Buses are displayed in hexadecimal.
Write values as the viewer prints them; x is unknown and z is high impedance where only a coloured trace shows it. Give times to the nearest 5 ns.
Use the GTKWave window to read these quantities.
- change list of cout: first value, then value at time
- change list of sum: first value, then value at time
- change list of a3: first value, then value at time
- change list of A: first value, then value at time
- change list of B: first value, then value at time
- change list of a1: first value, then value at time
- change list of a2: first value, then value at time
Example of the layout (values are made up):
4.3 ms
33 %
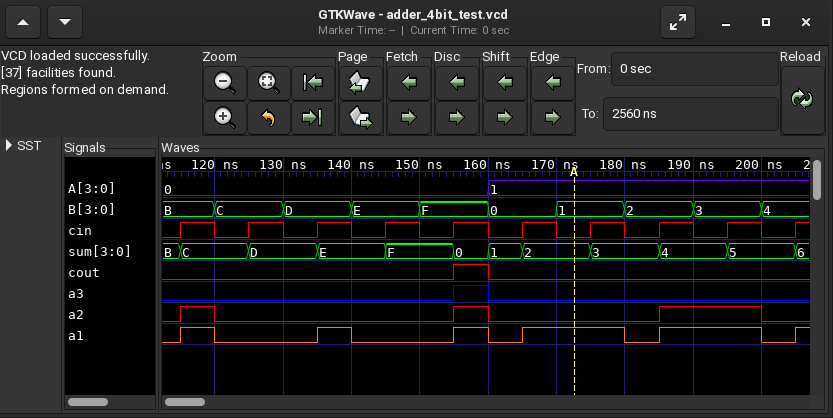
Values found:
0, 1 at 155 ns, 0 at 160 ns
B, C at 115 ns, D at 125 ns, E at 135 ns, F at 145 ns, 0 at 155 ns, 1 at 160 ns, 2 at 165 ns, 3 at 175 ns, 4 at 185 ns, 5 at 195 ns, 6 at 205 ns
0, 1 at 155 ns, 0 at 160 ns
0, 1 at 160 ns
B, C at 120 ns, D at 130 ns, E at 140 ns, F at 150 ns, 0 at 160 ns, 1 at 170 ns, 2 at 180 ns, 3 at 190 ns, 4 at 200 ns
0, 1 at 115 ns, 0 at 120 ns, 1 at 135 ns, 0 at 140 ns, 1 at 155 ns, 0 at 160 ns, 1 at 165 ns, 0 at 180 ns, 1 at 185 ns, 0 at 200 ns, 1 at 205 ns
0, 1 at 115 ns, 0 at 120 ns, 1 at 155 ns, 0 at 160 ns, 1 at 185 ns, 0 at 200 ns
